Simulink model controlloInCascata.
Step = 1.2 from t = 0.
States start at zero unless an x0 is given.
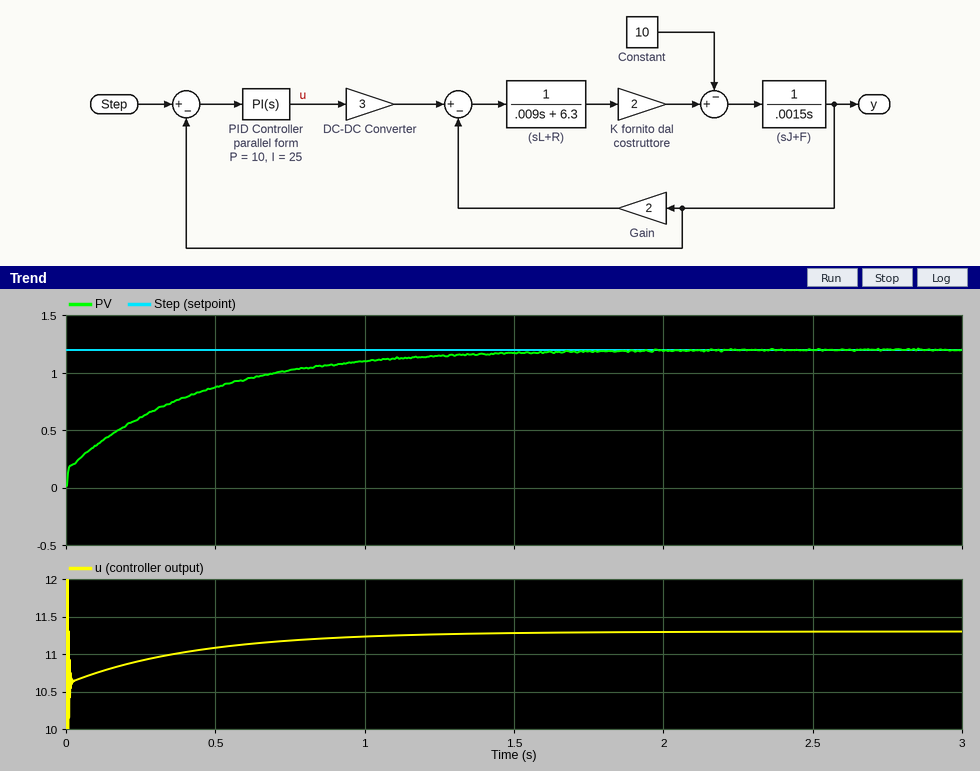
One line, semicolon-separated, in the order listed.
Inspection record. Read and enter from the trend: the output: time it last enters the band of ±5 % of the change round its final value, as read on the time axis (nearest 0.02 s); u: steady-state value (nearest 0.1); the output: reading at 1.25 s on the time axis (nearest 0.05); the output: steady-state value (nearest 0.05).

1.22 s; 11.3; 1.15; 1.20
